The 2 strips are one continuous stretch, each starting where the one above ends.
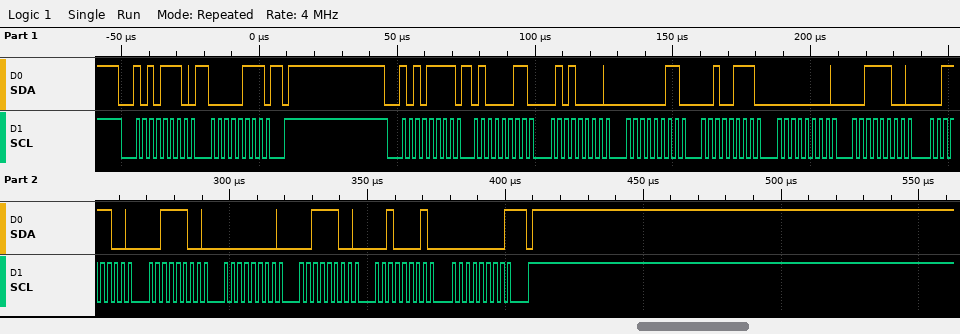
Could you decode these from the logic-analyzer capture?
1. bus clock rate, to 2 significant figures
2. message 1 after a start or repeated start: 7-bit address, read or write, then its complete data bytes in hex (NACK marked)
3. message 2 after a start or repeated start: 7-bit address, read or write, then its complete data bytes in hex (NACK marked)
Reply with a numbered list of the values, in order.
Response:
1. 400 kHz
2. 0x57 write: 07
3. 0x57 read: 43 50 03 27 00 3C 3C 3C 00 3C 21 00 NACK
